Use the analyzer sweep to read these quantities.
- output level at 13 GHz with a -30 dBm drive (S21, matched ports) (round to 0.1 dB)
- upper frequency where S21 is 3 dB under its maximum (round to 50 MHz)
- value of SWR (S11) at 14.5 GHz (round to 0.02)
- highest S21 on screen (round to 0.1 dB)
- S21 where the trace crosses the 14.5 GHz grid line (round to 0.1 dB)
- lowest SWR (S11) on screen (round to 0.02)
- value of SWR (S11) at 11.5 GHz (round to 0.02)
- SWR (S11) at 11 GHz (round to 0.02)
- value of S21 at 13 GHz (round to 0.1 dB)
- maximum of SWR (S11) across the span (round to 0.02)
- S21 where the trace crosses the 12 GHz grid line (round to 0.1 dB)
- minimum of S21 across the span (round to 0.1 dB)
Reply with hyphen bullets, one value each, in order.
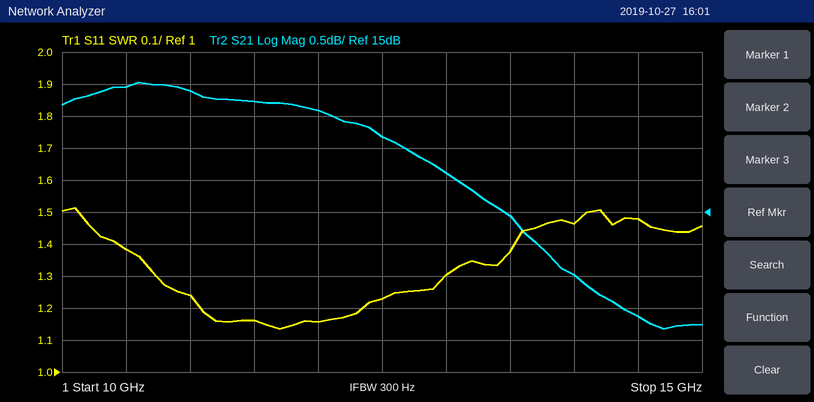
- -14.4 dBm
- 14.00 GHz
- 1.48
- 17.0 dB
- 13.4 dB
- 1.14
- 1.16
- 1.24
- 15.6 dB
- 1.52
- 16.6 dB
- 13.2 dB
